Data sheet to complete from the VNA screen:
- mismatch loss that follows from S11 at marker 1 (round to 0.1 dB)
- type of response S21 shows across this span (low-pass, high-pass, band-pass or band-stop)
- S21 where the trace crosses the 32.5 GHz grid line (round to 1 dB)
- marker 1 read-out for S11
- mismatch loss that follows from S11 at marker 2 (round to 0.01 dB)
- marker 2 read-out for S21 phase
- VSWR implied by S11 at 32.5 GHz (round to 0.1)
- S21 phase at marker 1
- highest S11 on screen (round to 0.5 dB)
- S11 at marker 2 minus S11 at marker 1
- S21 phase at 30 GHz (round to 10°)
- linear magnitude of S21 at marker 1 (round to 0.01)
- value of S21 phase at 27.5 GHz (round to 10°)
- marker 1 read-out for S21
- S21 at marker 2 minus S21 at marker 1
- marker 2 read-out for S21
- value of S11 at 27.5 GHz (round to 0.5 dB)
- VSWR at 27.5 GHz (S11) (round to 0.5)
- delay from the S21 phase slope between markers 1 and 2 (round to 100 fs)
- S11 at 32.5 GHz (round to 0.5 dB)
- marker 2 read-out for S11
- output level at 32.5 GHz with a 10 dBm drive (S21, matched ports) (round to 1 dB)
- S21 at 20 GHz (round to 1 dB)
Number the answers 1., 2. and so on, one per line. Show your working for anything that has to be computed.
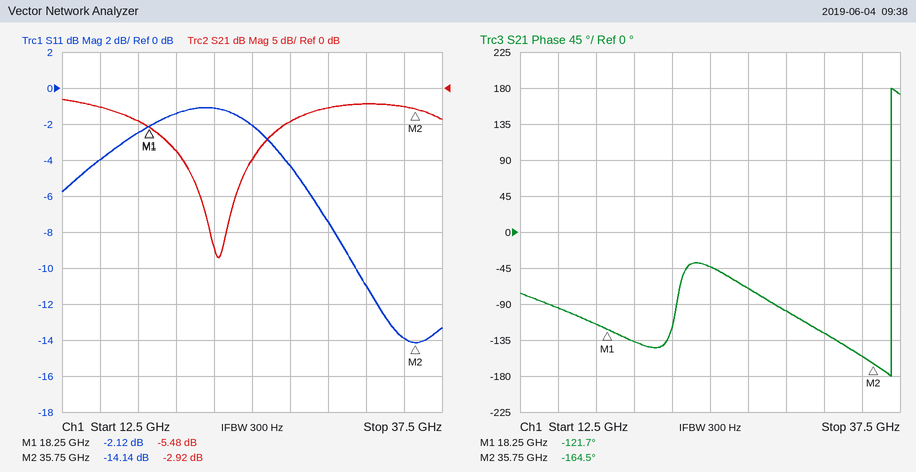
1. −10 log10(1 − 10^(-2.12/10)) ≈ 4.1 dB
2. band-stop
3. -2 dB
4. -2.12 dB
5. −10 log10(1 − 10^(-14.14/10)) ≈ 0.17 dB
6. -164.5°
7. |Γ| = 10^(-11/20) = 0.2818; VSWR = (1 + 0.2818)/(1 − 0.2818) ≈ 1.8
8. -121.7°
9. -1.0 dB
10. -14.14 − (-2.12) = -12.02 dB
11. -100°
12. 10^(-5.48/20) ≈ 0.53
13. -70°
14. -5.48 dB
15. -2.92 − (-5.48) = 2.56 dB
16. -2.92 dB
17. -4.5 dB
18. |Γ| = 10^(-4.5/20) = 0.5957; VSWR = (1 + 0.5957)/(1 − 0.5957) ≈ 4.0
19. −(-164.5° − (-121.7°))/(360° × 17.5 GHz) ≈ 6.8 ps
20. -11.0 dB
21. -14.14 dB
22. 10 dBm + (-2 dB) = 8 dBm
23. -9 dB
